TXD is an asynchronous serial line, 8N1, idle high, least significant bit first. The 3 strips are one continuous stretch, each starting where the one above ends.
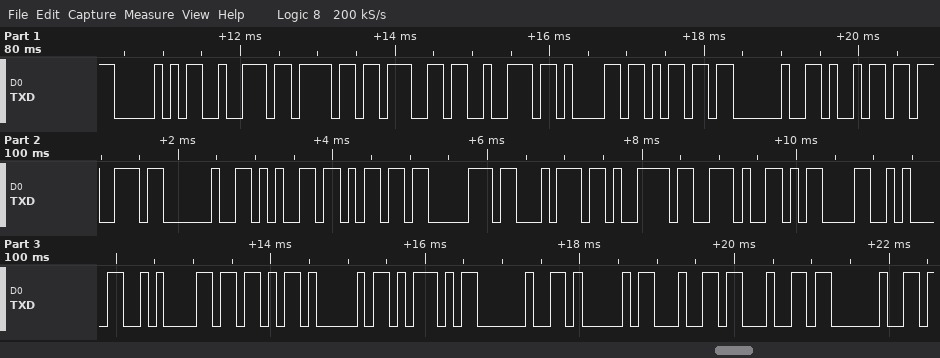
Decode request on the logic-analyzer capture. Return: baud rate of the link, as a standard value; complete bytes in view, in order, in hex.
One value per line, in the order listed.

9600 baud
50 72 6F 67 72 61 6D 20 69 73 20 65 6D 70 74 79 2E 0D 0A 0A 5B 41 5D 20 41 64 64 20
